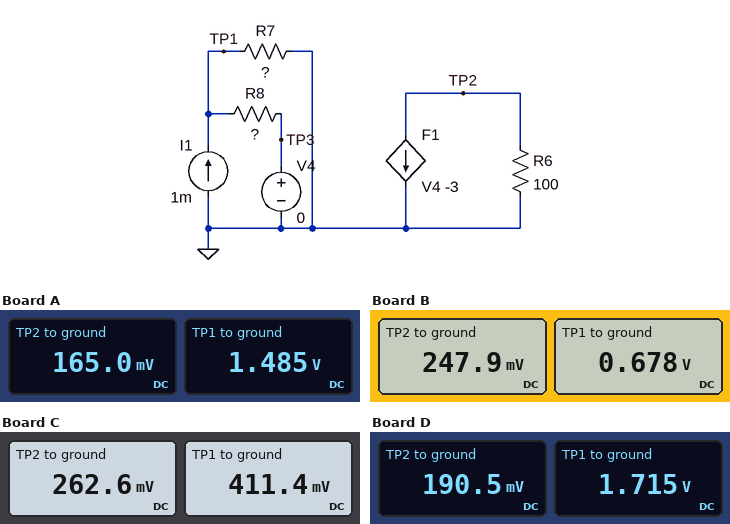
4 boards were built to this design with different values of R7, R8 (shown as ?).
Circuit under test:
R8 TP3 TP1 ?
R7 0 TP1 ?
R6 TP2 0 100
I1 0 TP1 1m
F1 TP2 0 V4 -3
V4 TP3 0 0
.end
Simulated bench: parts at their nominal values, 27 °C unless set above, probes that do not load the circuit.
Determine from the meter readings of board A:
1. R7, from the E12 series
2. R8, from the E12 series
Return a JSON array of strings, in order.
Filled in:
["3.3 kΩ", "2.7 kΩ"]
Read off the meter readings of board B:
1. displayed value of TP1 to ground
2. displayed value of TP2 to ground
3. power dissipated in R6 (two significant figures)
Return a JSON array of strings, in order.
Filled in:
["0.678 V", "247.9 mV", "610 µW"]
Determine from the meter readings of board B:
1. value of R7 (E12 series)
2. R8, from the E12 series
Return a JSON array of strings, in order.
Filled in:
["3.9 kΩ", "820 Ω"]
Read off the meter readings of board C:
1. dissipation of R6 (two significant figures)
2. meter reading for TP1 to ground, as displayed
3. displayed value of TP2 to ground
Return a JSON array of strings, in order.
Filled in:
["690 µW", "411.4 mV", "262.6 mV"]
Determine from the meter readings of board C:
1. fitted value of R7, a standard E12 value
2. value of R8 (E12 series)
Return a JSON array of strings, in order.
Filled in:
["3.3 kΩ", "470 Ω"]
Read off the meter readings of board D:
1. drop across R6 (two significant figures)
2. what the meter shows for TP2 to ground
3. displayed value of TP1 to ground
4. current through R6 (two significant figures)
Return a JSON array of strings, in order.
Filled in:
["190 mV", "190.5 mV", "1.715 V", "1.9 mA"]
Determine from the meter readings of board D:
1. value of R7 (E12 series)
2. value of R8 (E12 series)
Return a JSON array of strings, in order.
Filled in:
["4.7 kΩ", "2.7 kΩ"]
